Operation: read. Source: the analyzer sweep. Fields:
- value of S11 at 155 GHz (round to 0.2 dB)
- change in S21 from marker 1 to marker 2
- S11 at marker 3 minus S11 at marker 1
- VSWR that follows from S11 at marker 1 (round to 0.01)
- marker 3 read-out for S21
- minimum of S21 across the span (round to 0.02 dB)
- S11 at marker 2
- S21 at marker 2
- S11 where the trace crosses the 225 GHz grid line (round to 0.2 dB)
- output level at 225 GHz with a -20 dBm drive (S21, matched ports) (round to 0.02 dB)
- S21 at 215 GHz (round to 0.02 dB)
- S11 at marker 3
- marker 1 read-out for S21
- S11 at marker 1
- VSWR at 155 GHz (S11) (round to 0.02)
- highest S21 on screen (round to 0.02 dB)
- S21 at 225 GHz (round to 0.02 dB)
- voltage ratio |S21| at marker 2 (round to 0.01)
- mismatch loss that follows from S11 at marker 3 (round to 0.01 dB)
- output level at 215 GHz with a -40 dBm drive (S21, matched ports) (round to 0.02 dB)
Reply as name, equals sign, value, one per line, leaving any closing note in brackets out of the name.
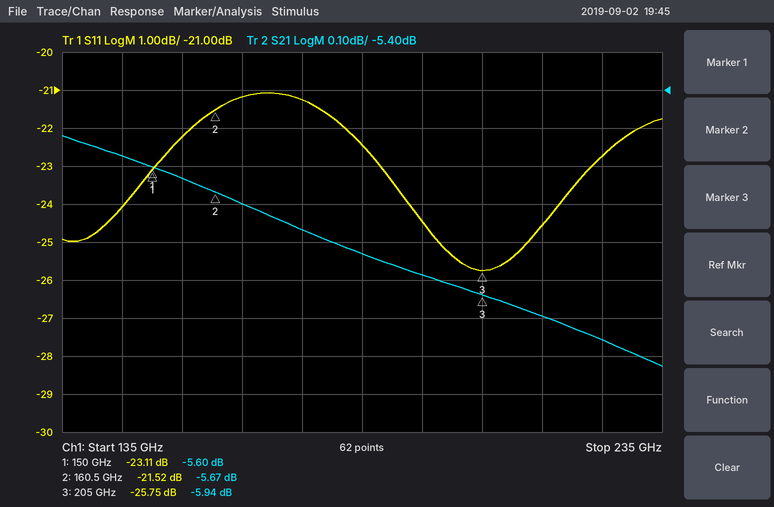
value of S11 at 155 GHz = -22.2 dB
change in S21 from marker 1 to marker 2 = -0.07 dB
S11 at marker 3 minus S11 at marker 1 = -2.64 dB
VSWR that follows from S11 at marker 1 = 1.15
marker 3 read-out for S21 = -5.94 dB
minimum of S21 across the span = -6.12 dB
S11 at marker 2 = -21.52 dB
S21 at marker 2 = -5.67 dB
S11 where the trace crosses the 225 GHz grid line = -22.8 dB
output level at 225 GHz with a -20 dBm drive (S21, matched ports) = -26.06 dBm
S21 at 215 GHz = -6.00 dB
S11 at marker 3 = -25.75 dB
marker 1 read-out for S21 = -5.60 dB
S11 at marker 1 = -23.11 dB
VSWR at 155 GHz (S11) = 1.16
highest S21 on screen = -5.52 dB
S21 at 225 GHz = -6.06 dB
voltage ratio |S21| at marker 2 = 0.52
mismatch loss that follows from S11 at marker 3 = 0.01 dB
output level at 215 GHz with a -40 dBm drive (S21, matched ports) = -46.00 dBm
